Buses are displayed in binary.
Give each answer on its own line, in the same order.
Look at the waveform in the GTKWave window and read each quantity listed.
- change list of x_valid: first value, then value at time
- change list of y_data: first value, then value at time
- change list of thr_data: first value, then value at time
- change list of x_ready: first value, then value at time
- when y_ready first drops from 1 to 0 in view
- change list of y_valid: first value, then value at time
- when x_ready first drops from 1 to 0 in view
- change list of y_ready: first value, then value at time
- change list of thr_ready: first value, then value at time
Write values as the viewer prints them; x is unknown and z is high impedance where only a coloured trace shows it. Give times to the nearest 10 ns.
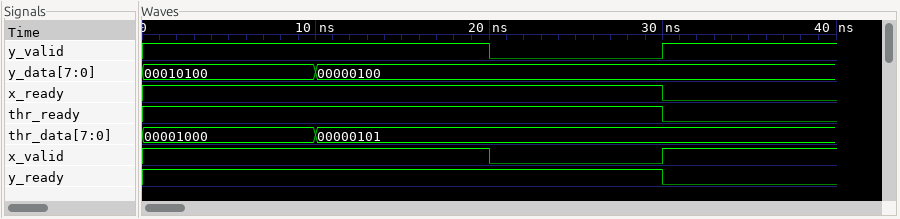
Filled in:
1, 0 at 20 ns, 1 at 30 ns
00010100, 00000100 at 10 ns
00001000, 00000101 at 10 ns
1, 0 at 30 ns
30 ns
1, 0 at 20 ns, 1 at 30 ns
30 ns
1, 0 at 30 ns
1, 0 at 30 ns
